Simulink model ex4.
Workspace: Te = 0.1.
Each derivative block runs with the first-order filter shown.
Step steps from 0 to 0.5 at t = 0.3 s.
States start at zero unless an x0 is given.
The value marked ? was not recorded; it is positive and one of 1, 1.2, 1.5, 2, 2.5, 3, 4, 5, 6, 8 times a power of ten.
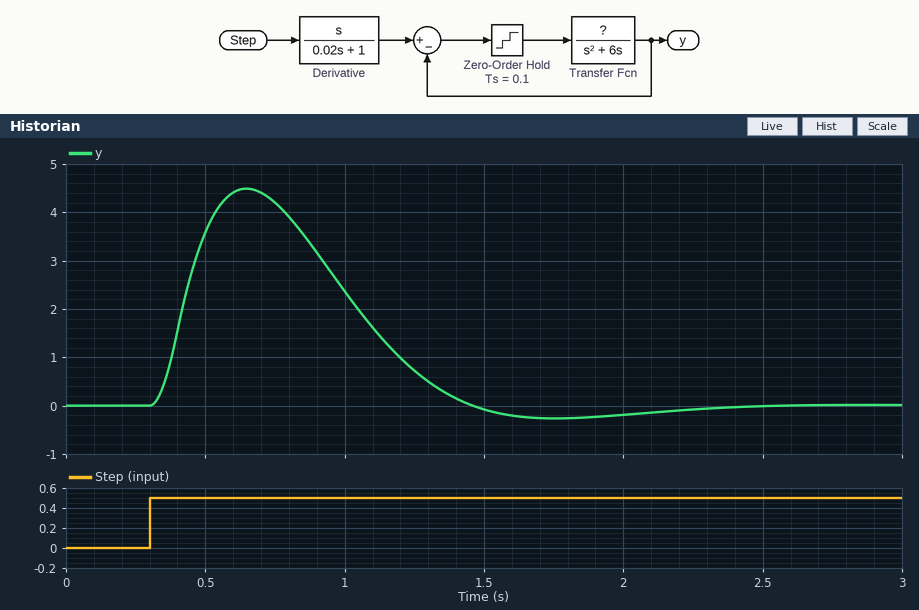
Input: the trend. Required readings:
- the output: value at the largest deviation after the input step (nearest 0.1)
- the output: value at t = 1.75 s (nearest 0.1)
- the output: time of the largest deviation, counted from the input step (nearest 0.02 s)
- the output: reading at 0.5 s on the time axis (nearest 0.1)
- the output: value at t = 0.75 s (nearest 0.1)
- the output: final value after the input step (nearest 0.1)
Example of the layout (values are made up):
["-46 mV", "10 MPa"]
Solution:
["4.5", "-0.3", "0.34 s", "3.6", "4.2", "0.0"]
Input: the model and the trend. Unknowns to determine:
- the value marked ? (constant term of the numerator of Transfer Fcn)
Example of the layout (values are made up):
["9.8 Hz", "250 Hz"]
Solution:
["15"]
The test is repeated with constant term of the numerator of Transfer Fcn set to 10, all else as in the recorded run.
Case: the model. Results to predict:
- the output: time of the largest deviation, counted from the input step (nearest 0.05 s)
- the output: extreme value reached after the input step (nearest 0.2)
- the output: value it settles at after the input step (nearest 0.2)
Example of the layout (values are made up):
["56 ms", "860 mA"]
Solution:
["0.40 s", "3.2", "0.0"]
